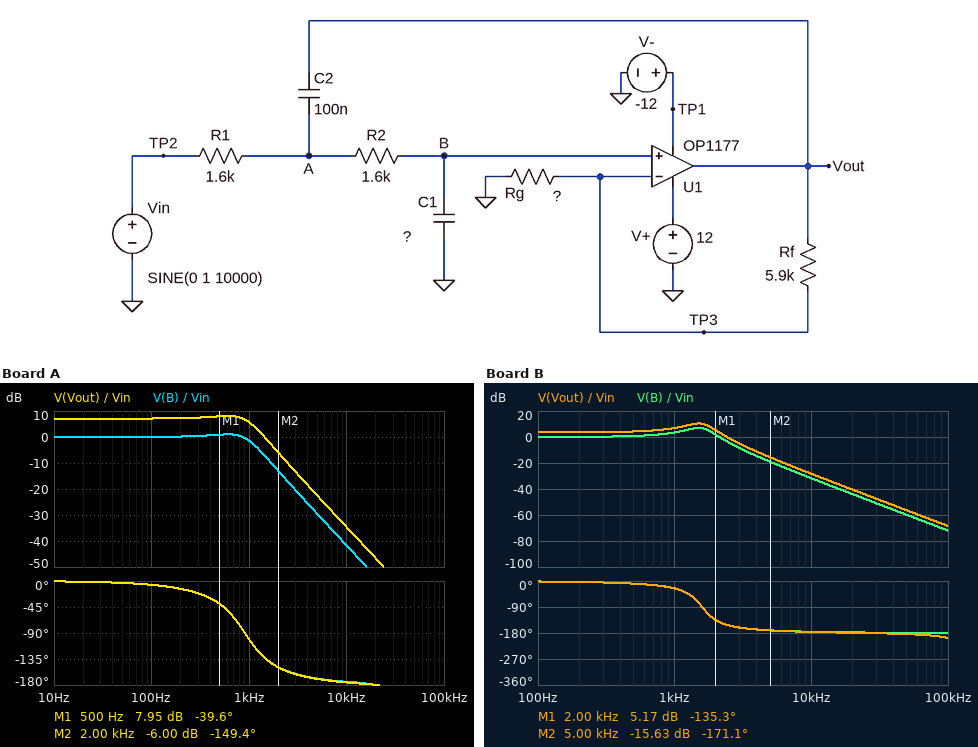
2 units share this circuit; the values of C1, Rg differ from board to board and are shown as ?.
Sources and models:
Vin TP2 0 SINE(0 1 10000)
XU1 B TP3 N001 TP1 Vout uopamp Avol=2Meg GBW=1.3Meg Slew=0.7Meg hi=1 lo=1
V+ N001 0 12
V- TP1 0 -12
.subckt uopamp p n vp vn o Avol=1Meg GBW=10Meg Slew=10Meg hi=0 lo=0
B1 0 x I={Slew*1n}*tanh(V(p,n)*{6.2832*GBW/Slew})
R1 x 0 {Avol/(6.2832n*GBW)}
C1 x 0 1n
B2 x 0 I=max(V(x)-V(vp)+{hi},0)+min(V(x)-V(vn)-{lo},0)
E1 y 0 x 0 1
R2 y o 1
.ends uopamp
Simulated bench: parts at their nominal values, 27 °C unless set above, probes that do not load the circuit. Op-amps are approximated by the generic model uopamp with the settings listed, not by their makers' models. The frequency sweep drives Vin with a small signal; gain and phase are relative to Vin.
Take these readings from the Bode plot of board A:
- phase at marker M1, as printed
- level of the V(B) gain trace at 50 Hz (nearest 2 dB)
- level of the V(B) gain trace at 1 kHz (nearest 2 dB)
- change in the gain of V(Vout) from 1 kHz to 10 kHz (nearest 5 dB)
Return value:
-39.6 deg
0 dB
-2 dB
-40 dB
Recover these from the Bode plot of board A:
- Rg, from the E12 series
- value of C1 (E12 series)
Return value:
4.7 kΩ
120 nF
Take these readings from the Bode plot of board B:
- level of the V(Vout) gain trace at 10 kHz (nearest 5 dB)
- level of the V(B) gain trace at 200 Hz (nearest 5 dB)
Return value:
-30 dB
0 dB
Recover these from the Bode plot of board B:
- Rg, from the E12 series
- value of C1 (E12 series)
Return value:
12 kΩ
39 nF
